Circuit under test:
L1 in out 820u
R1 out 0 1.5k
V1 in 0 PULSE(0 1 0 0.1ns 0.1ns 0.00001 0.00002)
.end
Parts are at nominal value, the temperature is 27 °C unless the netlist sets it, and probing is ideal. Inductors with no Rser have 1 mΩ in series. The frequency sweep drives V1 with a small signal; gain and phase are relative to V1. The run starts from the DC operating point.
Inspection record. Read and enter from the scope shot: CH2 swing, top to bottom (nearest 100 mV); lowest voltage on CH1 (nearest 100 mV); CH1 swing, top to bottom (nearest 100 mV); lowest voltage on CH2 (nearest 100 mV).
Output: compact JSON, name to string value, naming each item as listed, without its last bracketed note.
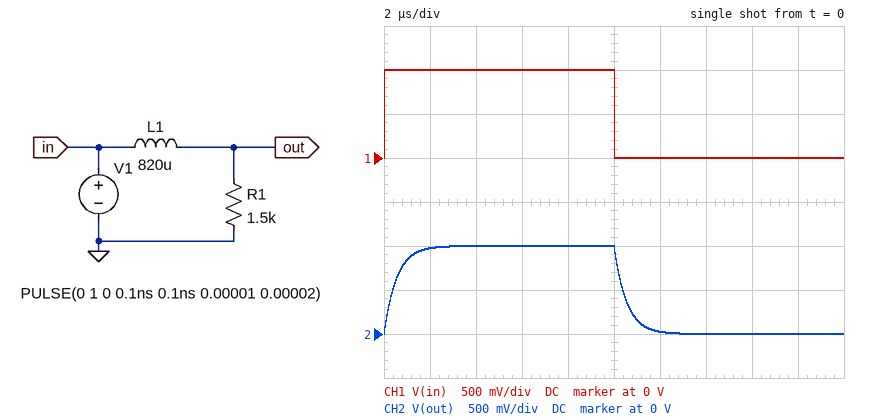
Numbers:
{"CH2 swing, top to bottom": "1.0 V", "lowest voltage on CH1": "0 V", "CH1 swing, top to bottom": "1.0 V", "lowest voltage on CH2": "0 V"}
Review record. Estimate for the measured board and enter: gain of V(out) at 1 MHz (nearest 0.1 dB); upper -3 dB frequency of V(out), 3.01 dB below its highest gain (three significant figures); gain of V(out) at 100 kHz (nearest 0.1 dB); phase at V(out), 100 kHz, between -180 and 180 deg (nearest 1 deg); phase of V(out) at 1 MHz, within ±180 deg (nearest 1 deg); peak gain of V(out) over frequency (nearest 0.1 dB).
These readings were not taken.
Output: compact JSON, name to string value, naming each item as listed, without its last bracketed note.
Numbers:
{"gain of V(out) at 1 MHz": "-11.1 dB", "upper -3 dB frequency of V(out), 3.01 dB below its highest gain": "291 kHz", "gain of V(out) at 100 kHz": "-0.5 dB", "phase at V(out), 100 kHz, between -180 and 180 deg": "-19 deg", "phase of V(out) at 1 MHz, within ±180 deg": "-74 deg", "peak gain of V(out) over frequency": "0 dB"}
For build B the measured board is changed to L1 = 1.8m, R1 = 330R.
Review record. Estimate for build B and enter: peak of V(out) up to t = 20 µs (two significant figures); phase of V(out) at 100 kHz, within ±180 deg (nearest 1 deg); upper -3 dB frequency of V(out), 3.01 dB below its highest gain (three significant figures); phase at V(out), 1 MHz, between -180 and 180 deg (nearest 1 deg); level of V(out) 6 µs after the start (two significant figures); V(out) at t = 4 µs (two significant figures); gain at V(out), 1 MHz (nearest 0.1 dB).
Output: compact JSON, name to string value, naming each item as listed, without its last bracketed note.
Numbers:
{"peak of V(out) up to t = 20 µs": "840 mV", "phase of V(out) at 100 kHz, within ±180 deg": "-74 deg", "upper -3 dB frequency of V(out), 3.01 dB below its highest gain": "29.2 kHz", "phase at V(out), 1 MHz, between -180 and 180 deg": "-88 deg", "level of V(out) 6 µs after the start": "670 mV", "V(out) at t = 4 µs": "520 mV", "gain at V(out), 1 MHz": "-30.7 dB"}
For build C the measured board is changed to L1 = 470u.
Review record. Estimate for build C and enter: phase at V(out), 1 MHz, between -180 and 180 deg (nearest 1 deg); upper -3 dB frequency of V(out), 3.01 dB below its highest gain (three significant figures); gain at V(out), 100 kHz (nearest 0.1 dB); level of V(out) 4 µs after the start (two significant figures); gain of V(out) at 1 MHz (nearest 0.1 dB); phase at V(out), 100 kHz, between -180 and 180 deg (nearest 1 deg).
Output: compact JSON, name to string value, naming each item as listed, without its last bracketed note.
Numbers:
{"phase at V(out), 1 MHz, between -180 and 180 deg": "-63 deg", "upper -3 dB frequency of V(out), 3.01 dB below its highest gain": "508 kHz", "gain at V(out), 100 kHz": "-0.2 dB", "level of V(out) 4 µs after the start": "1.0 V", "gain of V(out) at 1 MHz": "-6.9 dB", "phase at V(out), 100 kHz, between -180 and 180 deg": "-11 deg"}
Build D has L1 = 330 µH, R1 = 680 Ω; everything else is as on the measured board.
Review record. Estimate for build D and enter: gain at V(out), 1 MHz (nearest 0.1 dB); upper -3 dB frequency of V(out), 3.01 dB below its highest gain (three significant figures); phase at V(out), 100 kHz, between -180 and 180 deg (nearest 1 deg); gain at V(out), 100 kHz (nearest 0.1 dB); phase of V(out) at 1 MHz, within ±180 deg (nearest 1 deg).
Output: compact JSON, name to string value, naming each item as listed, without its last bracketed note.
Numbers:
{"gain at V(out), 1 MHz": "-10.1 dB", "upper -3 dB frequency of V(out), 3.01 dB below its highest gain": "328 kHz", "phase at V(out), 100 kHz, between -180 and 180 deg": "-17 deg", "gain at V(out), 100 kHz": "-0.4 dB", "phase of V(out) at 1 MHz, within ±180 deg": "-72 deg"}
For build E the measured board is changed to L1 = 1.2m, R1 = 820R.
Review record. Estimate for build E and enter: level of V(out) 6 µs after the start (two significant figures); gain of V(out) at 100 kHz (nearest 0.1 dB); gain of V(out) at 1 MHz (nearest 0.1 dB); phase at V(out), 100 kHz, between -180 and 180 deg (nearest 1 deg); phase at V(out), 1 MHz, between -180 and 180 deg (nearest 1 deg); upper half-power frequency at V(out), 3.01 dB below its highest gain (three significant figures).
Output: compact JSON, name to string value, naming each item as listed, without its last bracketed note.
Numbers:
{"level of V(out) 6 µs after the start": "980 mV", "gain of V(out) at 100 kHz": "-2.7 dB", "gain of V(out) at 1 MHz": "-19.3 dB", "phase at V(out), 100 kHz, between -180 and 180 deg": "-43 deg", "phase at V(out), 1 MHz, between -180 and 180 deg": "-84 deg", "upper half-power frequency at V(out), 3.01 dB below its highest gain": "109 kHz"}
